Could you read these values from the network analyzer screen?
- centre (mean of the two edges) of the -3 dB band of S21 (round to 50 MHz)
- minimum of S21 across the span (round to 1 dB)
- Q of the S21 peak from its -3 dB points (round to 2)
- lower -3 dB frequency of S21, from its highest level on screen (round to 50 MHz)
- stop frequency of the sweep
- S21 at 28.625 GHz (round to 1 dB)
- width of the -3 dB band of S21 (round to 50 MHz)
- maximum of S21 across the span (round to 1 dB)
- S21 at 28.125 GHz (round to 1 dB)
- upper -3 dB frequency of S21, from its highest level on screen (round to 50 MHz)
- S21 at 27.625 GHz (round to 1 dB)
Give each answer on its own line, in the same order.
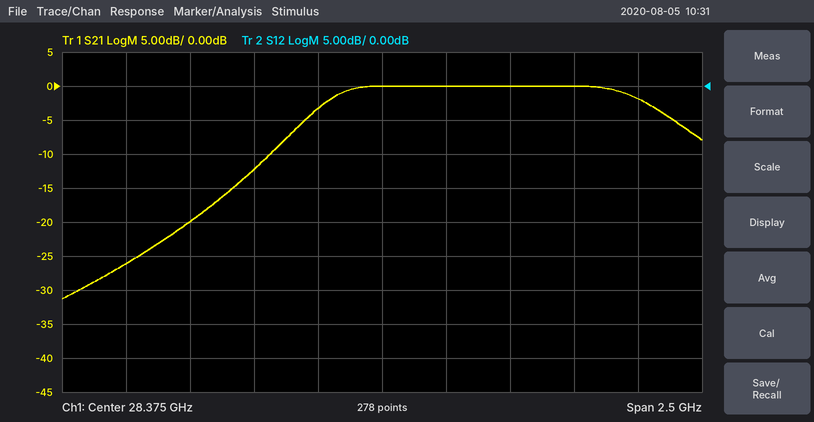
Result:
28.80 GHz
-31 dB
22
28.15 GHz
29.625 GHz
0 dB
1.30 GHz
0 dB
-3 dB
29.45 GHz
-20 dB
